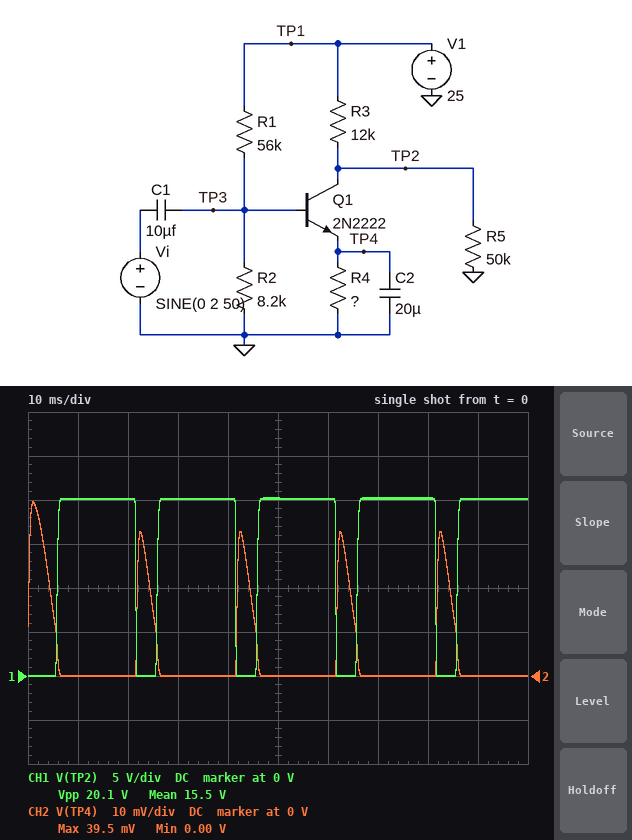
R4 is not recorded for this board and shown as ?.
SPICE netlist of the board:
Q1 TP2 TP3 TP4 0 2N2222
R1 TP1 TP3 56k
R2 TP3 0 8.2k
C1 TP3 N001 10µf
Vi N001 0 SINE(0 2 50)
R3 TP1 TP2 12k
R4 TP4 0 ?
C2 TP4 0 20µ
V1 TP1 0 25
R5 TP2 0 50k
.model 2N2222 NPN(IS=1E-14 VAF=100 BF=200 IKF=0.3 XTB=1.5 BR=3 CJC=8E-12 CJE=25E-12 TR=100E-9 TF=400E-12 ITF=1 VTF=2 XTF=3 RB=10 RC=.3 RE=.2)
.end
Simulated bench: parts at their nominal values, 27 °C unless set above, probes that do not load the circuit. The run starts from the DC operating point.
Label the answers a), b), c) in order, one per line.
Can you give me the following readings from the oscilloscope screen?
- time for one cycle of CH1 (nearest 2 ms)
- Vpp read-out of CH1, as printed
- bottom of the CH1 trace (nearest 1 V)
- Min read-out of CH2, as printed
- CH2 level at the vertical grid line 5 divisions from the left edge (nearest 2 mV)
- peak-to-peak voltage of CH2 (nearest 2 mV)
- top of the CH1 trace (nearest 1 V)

a) 20 ms
b) 20.1 V
c) 0 V
d) 0.00 V
e) 0 V
f) 40 mV
g) 20 V
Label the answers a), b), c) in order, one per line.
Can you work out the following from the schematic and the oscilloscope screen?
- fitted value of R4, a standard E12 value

a) 4.7 Ω
